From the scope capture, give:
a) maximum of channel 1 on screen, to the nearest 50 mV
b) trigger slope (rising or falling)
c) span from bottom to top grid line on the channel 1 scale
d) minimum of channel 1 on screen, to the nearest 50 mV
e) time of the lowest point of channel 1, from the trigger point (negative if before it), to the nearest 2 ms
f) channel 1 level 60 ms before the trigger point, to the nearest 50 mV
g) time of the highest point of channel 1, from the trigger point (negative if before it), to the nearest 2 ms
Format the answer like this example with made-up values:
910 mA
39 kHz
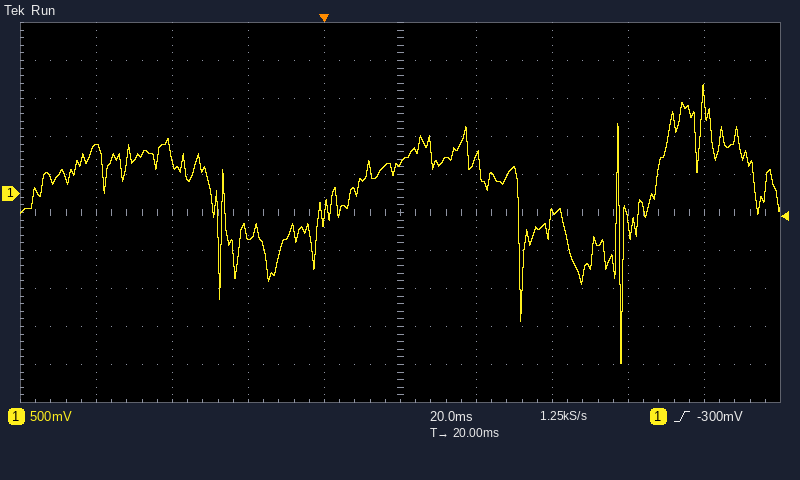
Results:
1.45 V
rising
5 V
-2.25 V
+78 ms
600 mV
+100 ms
